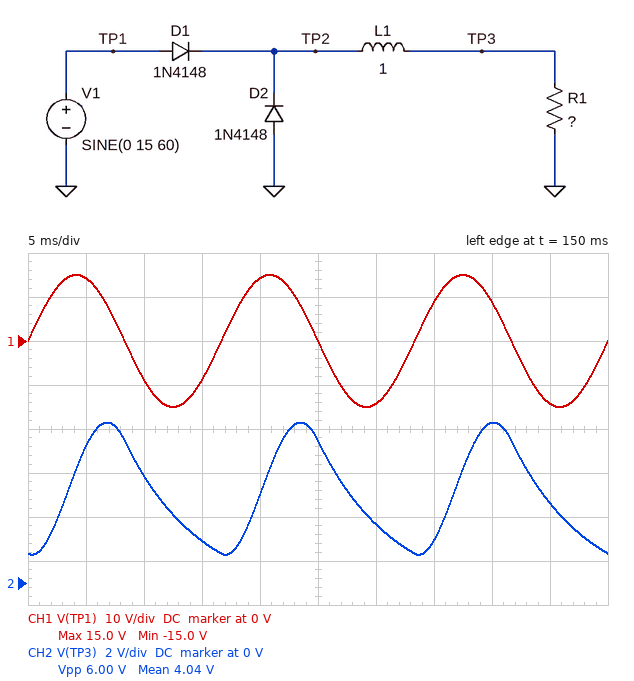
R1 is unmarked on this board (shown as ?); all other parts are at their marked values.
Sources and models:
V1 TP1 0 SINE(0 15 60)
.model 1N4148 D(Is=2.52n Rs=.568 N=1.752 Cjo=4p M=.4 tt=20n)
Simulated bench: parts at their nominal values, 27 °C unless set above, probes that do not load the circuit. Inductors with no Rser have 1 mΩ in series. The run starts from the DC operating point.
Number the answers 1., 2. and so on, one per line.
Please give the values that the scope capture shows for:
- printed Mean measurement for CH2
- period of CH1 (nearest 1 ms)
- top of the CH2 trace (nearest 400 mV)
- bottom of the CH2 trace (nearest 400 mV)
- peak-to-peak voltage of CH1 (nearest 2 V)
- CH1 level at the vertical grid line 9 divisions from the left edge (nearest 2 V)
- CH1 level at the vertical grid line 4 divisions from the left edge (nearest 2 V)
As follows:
1. 4.04 V
2. 17 ms
3. 7.2 V
4. 1.2 V
5. 30 V
6. -14 V
7. 14 V
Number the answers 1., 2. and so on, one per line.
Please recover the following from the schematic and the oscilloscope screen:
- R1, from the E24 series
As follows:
1. 150 Ω
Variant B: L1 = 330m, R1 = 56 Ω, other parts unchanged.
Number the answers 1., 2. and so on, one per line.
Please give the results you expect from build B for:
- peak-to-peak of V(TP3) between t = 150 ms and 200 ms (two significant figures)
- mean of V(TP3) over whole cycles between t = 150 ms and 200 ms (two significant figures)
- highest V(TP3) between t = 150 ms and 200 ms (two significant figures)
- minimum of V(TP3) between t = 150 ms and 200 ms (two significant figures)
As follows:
1. 6.6 V
2. 4.0 V
3. 7.6 V
4. 970 mV
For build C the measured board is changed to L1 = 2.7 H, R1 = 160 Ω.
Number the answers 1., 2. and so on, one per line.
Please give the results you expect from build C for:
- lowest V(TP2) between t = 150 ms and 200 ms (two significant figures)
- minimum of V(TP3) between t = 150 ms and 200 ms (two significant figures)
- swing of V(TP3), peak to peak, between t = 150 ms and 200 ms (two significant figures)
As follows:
1. -760 mV
2. 2.8 V
3. 2.6 V
